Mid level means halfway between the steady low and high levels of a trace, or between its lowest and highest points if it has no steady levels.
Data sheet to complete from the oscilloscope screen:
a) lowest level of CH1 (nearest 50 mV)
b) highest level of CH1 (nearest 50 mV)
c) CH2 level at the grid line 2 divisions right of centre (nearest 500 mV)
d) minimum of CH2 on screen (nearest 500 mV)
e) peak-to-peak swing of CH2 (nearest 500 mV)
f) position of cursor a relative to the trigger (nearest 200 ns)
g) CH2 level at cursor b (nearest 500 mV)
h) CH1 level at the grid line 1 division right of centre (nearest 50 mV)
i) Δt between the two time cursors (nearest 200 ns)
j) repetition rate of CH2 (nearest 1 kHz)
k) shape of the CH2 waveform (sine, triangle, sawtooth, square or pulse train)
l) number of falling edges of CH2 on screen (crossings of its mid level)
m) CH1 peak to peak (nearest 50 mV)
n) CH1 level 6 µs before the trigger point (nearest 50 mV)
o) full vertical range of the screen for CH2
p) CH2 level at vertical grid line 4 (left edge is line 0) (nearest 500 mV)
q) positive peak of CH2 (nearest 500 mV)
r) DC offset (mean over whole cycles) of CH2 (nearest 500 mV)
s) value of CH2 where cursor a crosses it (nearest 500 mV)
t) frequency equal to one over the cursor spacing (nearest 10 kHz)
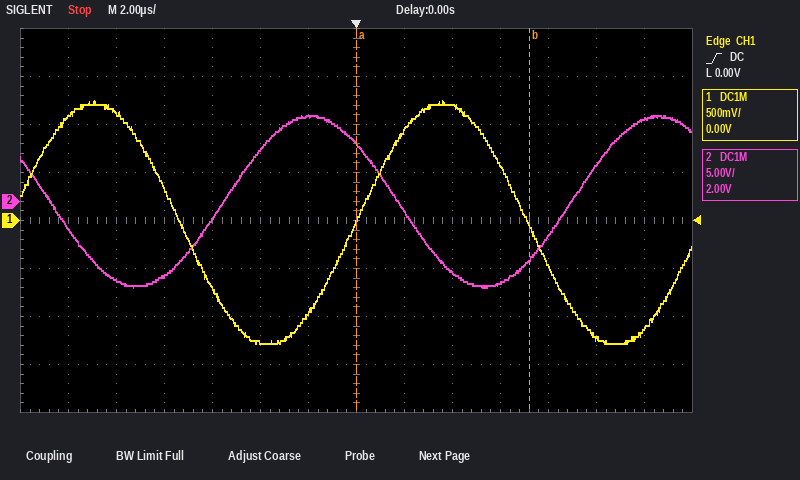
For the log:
-1.30 V
1.25 V
-7.5 V
-9.0 V
18.0 V
0.0 µs
-6.0 V
950 mV
7.2 µs
69 kHz
sine
2
2.55 V
-700 mV
40 V
-2.0 V
9.0 V
0.0 V
6.0 V
140 kHz
